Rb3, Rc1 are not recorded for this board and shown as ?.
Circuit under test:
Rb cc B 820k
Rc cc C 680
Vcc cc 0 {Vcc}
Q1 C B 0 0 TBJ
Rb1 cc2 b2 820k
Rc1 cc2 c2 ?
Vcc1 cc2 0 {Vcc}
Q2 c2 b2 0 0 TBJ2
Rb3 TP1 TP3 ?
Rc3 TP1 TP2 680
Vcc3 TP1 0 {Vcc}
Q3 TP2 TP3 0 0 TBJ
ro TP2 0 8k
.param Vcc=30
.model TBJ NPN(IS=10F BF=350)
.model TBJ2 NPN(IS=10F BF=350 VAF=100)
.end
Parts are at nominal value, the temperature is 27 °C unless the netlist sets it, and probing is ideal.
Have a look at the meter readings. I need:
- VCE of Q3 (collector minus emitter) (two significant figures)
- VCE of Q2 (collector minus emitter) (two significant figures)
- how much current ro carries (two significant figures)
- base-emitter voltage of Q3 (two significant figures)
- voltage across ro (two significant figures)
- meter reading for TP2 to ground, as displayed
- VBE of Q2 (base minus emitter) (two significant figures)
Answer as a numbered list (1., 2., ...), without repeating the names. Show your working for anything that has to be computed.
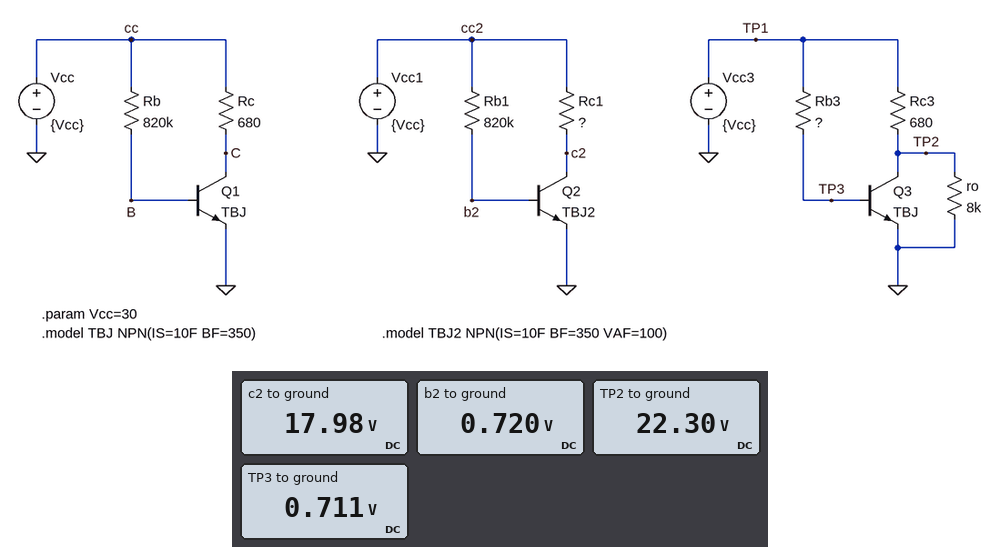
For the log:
1. 22.3 V = 22 V
2. 17.98 V = 18 V
3. (22.3 V) / 8 kΩ = 2.8 mA
4. 711 mV = 710 mV
5. 22.3 V = 22 V
6. 22.30 V
7. 720 mV = 720 mV
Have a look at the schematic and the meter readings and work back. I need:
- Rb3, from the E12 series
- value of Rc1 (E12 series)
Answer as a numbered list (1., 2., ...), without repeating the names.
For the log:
1. 1.2 MΩ
2. 820 Ω
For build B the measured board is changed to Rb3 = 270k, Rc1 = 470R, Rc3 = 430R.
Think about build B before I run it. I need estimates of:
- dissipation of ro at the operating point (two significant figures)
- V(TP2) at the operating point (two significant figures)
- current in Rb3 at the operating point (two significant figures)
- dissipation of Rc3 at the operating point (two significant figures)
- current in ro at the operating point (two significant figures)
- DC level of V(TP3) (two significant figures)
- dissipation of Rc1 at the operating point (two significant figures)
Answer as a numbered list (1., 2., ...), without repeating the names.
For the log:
1. 21 mW
2. 13 V
3. 110 µA
4. 670 mW
5. 1.6 mA
6. 750 mV
7. 110 mW
